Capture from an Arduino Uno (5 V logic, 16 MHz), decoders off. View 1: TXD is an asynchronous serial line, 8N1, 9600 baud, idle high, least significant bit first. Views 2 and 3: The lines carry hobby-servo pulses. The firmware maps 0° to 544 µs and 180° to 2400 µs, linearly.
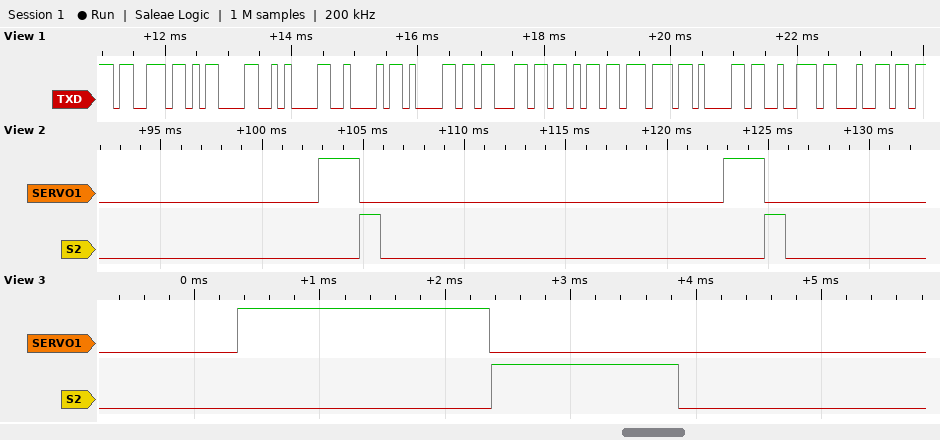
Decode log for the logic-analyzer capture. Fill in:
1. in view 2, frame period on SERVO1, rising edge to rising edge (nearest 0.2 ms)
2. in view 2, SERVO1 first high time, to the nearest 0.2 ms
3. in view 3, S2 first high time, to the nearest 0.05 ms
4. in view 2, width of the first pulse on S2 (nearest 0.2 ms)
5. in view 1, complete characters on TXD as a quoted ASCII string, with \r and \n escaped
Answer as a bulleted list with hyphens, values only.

- 20.0 ms
- 2.0 ms
- 1.50 ms
- 1.0 ms
- "s\r\nBackward"
